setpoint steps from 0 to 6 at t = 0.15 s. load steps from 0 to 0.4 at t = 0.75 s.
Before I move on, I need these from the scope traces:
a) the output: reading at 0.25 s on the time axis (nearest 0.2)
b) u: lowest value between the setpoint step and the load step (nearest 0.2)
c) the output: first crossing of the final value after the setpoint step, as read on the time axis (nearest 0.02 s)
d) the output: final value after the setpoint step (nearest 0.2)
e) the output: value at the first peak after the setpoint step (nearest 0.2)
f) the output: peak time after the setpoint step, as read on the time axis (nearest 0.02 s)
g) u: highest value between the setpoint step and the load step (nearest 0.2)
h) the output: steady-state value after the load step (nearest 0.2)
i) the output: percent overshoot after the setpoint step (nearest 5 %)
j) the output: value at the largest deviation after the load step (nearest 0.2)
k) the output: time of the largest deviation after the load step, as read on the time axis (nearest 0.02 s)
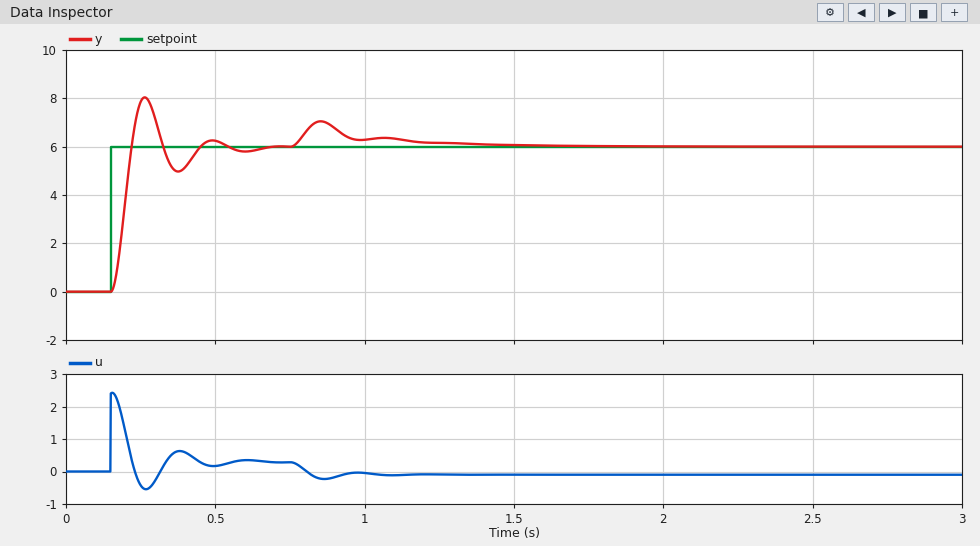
7.8
-0.6
0.22 s
6.0
8.0
0.26 s
2.4
6.0
35 %
7.0
0.86 s
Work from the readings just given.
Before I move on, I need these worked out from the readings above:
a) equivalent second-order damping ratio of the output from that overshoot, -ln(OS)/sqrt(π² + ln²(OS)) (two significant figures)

0.32
